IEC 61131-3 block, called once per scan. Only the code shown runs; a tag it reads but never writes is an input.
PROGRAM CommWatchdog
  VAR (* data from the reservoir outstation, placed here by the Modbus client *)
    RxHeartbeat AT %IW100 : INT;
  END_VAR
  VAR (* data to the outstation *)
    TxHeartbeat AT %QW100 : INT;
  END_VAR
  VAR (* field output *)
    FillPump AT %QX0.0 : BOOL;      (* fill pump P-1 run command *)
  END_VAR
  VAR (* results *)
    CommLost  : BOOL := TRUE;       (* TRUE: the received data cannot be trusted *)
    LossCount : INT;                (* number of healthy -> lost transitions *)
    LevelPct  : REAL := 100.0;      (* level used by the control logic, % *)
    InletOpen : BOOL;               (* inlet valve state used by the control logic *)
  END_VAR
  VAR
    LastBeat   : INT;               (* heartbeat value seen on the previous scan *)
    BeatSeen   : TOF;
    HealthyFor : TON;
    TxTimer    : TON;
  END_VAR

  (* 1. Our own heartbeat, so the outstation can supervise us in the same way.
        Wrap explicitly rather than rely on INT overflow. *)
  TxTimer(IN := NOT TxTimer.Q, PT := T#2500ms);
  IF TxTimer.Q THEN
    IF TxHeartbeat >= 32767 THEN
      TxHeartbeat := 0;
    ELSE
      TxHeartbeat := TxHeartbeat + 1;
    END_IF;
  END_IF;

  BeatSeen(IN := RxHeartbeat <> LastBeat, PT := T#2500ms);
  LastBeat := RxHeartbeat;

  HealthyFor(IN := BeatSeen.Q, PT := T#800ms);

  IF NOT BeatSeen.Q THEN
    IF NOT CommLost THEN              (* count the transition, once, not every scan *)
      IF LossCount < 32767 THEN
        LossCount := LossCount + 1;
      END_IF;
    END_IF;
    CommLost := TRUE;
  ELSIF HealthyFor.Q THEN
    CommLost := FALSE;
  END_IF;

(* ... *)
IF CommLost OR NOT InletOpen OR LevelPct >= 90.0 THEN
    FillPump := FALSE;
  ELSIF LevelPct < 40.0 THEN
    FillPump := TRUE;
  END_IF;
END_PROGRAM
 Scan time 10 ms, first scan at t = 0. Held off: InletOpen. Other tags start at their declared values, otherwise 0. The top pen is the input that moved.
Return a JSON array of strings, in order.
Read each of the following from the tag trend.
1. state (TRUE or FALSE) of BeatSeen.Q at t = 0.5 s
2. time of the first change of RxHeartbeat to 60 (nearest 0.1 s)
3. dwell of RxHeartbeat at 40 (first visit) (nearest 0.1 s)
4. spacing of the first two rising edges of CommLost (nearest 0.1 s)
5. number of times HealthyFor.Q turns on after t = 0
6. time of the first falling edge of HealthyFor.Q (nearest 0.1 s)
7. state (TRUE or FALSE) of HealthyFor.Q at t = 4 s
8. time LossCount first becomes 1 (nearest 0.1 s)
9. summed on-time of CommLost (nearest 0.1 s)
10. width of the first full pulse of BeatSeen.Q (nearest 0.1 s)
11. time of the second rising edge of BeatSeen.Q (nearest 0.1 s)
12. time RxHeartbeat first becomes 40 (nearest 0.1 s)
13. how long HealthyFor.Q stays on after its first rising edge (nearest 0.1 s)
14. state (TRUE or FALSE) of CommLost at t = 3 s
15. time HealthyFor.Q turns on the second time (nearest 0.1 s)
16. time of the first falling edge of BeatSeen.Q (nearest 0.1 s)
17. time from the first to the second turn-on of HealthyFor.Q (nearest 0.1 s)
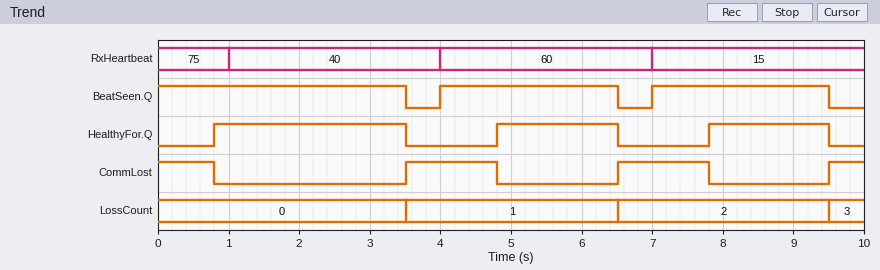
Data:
["TRUE", "4.0 s", "3.0 s", "3.0 s", "3", "3.5 s", "FALSE", "3.5 s", "3.9 s", "2.5 s", "7.0 s", "1.0 s", "2.7 s", "FALSE", "4.8 s", "3.5 s", "4.0 s"]
